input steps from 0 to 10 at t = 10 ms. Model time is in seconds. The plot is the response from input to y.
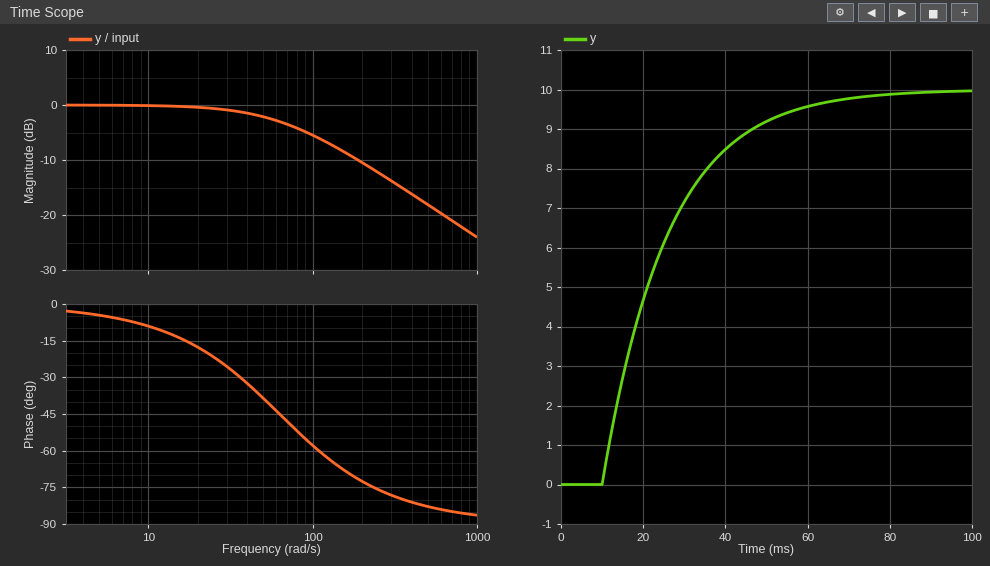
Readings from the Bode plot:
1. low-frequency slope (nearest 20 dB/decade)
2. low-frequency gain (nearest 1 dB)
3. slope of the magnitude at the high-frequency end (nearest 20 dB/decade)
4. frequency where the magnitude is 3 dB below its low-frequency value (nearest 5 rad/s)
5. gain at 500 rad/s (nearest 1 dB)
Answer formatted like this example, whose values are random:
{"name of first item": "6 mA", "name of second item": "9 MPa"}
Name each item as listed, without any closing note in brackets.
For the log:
{"low-frequency slope": "0 dB/decade", "low-frequency gain": "0 dB", "slope of the magnitude at the high-frequency end": "-20 dB/decade", "frequency where the magnitude is 3 dB below its low-frequency value": "65 rad/s", "gain at 500 rad/s": "-18 dB"}
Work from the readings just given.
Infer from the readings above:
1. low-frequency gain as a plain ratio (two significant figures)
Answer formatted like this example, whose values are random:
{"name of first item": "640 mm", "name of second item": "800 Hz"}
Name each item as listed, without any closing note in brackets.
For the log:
{"low-frequency gain as a plain ratio": "1.0"}
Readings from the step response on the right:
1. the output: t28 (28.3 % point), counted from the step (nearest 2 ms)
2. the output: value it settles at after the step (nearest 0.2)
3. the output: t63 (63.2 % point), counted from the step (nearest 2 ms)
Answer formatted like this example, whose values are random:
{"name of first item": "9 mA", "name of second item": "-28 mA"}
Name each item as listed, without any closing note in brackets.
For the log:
{"the output: t28 (28.3 % point), counted from the step": "6 ms", "the output: value it settles at after the step": "10.0", "the output: t63 (63.2 % point), counted from the step": "16 ms"}
